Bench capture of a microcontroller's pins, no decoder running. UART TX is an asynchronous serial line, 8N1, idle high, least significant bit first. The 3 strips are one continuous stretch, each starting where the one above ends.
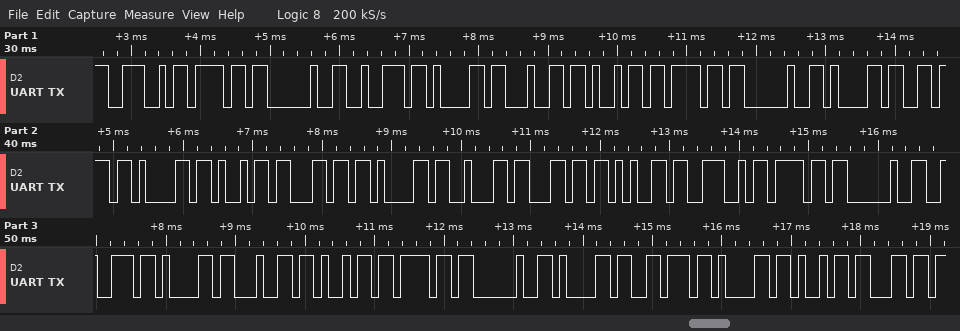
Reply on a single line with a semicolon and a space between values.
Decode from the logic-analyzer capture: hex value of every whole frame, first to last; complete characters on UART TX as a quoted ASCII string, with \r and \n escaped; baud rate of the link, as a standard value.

0x4E 0x6F 0x20 0x72 0x61 0x64 0x69 0x6F 0x20 0x61 0x76 0x61 0x69 0x6C 0x61 0x62 0x6C 0x65 0x4E 0x6F 0x20 0x72 0x61 0x64 0x69 0x6F 0x20 0x61 0x76 0x61 0x69 0x6C; "No radio availableNo radio avail"; 9600 baud
